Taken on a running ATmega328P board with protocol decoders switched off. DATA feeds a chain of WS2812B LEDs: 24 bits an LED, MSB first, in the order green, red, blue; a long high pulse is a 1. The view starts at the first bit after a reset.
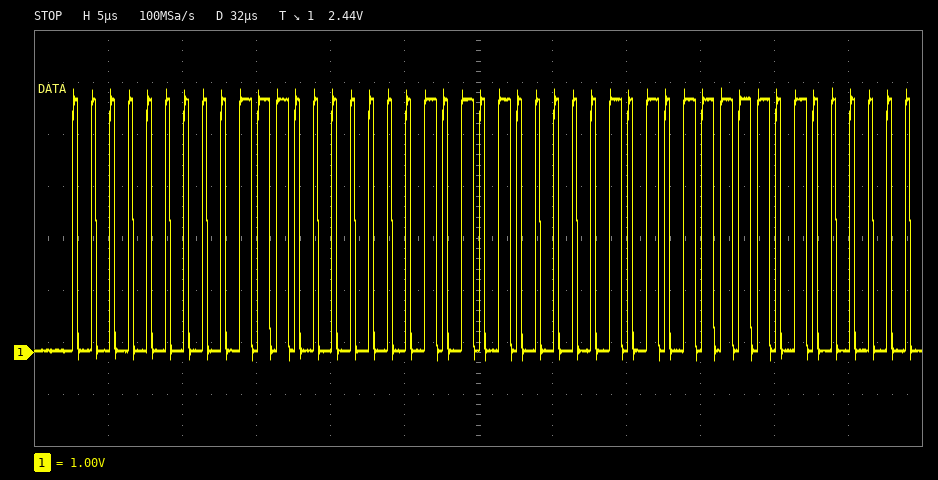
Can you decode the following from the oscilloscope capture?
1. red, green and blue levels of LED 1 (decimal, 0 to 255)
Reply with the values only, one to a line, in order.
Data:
112, 0, 21
